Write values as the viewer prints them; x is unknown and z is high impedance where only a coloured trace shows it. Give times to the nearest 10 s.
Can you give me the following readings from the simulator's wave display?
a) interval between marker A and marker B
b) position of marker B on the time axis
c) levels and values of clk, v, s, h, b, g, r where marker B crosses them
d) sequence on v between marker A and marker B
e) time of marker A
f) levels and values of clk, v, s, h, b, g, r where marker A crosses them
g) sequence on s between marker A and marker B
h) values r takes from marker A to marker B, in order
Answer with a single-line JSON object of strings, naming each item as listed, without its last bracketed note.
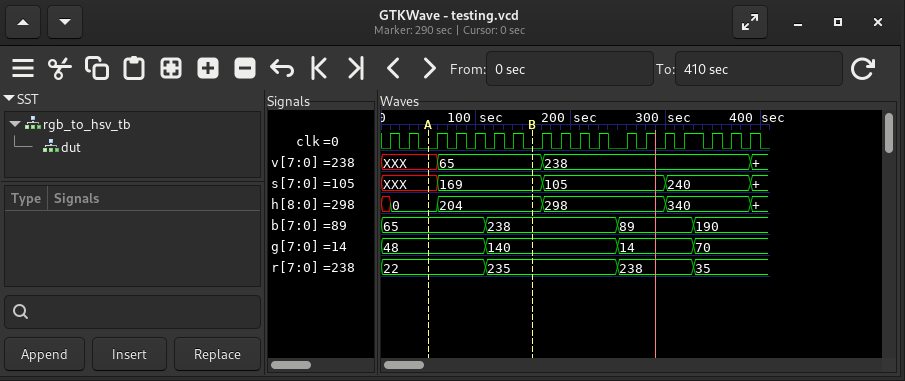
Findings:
{"interval between marker A and marker B": "110 s", "position of marker B on the time axis": "160 s", "levels and values of clk, v, s, h, b, g, r where marker B crosses them": "clk=0, v=65, s=169, h=204, b=238, g=140, r=235", "sequence on v between marker A and marker B": "XXX, 65", "time of marker A": "50 s", "levels and values of clk, v, s, h, b, g, r where marker A crosses them": "clk=0, v=XXX, s=XXX, h=0, b=65, g=48, r=22", "sequence on s between marker A and marker B": "XXX, 169", "values r takes from marker A to marker B, in order": "22, 235"}
